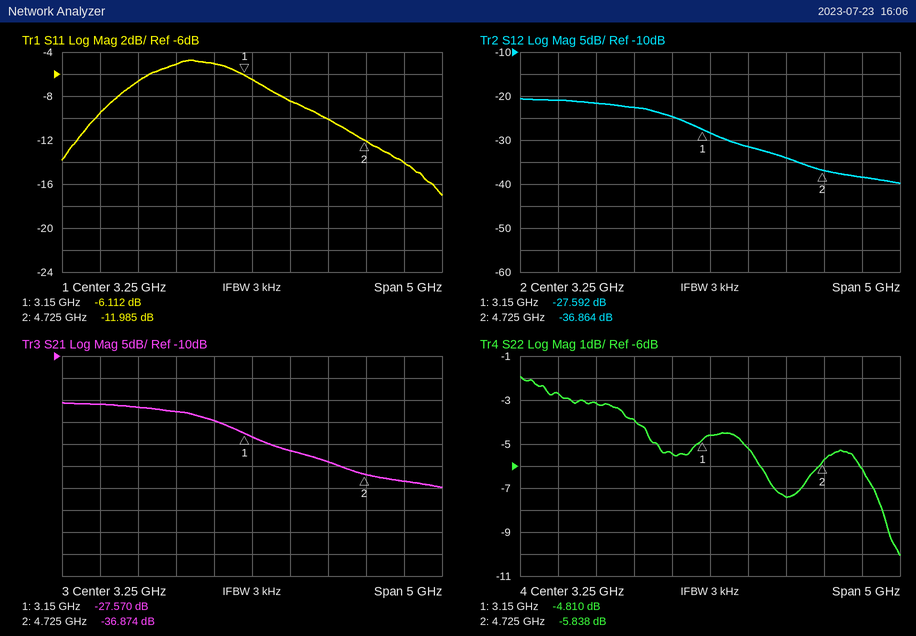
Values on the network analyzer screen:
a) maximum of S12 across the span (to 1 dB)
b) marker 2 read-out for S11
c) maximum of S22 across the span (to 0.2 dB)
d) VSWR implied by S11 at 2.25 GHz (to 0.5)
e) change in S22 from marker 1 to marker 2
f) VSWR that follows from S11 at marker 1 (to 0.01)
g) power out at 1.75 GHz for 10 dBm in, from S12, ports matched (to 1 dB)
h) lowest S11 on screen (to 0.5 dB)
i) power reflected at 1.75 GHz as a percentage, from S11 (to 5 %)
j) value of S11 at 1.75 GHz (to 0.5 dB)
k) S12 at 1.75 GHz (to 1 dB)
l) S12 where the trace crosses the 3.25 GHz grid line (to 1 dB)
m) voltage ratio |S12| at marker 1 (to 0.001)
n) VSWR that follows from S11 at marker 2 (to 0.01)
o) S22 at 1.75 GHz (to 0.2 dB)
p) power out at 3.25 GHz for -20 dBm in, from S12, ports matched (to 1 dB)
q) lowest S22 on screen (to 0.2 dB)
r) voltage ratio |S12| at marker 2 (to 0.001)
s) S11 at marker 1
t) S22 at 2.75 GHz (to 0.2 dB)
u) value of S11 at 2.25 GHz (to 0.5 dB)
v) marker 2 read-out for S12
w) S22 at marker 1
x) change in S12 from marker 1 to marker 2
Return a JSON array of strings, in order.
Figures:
["-21 dB", "-11.985 dB", "-2.0 dB", "3.5", "-1.028 dB", "2.96", "-12 dBm", "-17.0 dB", "20 %", "-6.5 dB", "-22 dB", "-28 dB", "0.042", "1.67", "-3.2 dB", "-48 dBm", "-10.0 dB", "0.014", "-6.112 dB", "-5.4 dB", "-5.0 dB", "-36.864 dB", "-4.810 dB", "-9.272 dB"]
